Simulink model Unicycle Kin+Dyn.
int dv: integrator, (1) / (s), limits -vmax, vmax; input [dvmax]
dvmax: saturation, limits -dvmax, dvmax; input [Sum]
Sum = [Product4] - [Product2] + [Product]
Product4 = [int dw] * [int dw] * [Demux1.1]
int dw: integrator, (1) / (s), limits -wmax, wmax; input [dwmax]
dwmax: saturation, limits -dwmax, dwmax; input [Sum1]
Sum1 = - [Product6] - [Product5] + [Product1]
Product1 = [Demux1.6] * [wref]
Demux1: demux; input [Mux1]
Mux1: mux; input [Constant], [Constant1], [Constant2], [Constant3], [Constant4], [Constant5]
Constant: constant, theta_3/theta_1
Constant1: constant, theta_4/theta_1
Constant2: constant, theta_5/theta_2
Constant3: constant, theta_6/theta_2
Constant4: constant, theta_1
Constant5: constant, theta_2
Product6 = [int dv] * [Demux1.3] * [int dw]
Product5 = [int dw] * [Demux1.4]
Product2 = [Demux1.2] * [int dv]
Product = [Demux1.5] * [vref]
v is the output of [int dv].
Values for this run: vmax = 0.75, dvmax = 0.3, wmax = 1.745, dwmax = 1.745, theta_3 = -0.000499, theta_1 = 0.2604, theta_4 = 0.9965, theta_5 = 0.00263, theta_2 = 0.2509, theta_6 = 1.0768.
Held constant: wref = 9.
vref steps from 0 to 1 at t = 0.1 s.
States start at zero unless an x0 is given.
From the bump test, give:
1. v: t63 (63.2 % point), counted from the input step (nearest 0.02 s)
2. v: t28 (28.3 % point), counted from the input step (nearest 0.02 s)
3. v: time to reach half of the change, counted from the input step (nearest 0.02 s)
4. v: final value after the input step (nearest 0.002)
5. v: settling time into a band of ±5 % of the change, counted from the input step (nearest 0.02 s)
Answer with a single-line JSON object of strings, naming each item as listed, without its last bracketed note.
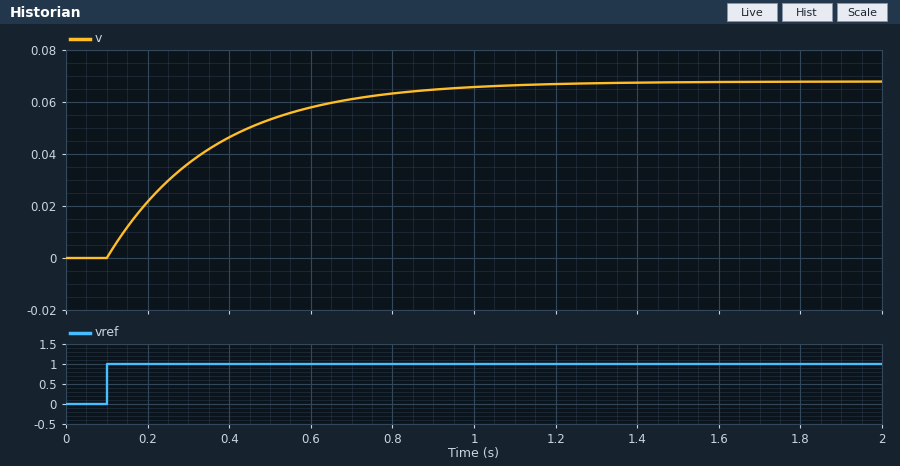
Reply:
{"v: t63 (63.2 % point), counted from the input step": "0.26 s", "v: t28 (28.3 % point), counted from the input step": "0.08 s", "v: time to reach half of the change, counted from the input step": "0.18 s", "v: final value after the input step": "0.068", "v: settling time into a band of ±5 % of the change, counted from the input step": "0.78 s"}
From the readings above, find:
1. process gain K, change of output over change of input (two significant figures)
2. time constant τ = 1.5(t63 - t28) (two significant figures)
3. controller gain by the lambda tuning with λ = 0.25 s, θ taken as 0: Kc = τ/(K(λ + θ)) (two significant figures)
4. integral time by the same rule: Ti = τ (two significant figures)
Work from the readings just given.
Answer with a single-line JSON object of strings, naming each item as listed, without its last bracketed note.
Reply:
{"process gain K, change of output over change of input": "0.068", "time constant τ = 1.5(t63 - t28)": "0.27 s", "controller gain by the lambda tuning with λ = 0.25 s, θ taken as 0: Kc = τ/(K(λ + θ))": "16", "integral time by the same rule: Ti = τ": "0.27 s"}
